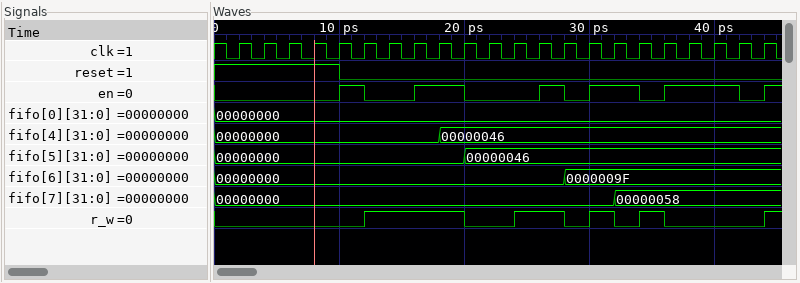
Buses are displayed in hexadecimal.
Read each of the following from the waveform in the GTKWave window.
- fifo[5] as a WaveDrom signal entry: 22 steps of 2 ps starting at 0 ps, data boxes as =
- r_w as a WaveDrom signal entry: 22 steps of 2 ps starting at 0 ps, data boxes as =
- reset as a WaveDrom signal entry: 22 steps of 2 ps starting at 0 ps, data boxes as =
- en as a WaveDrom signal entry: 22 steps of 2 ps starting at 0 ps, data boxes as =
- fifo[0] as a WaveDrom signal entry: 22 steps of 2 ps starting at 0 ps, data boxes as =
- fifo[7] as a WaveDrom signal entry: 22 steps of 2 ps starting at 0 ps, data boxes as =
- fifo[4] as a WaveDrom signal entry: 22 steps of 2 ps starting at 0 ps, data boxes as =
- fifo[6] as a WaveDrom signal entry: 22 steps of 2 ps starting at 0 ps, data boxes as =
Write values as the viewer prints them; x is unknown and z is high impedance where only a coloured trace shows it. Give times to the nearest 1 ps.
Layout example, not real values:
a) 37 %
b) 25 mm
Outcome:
a) {name: 'fifo[5]', wave: '=.........=...........', data: '00000000 00000046'}
b) {name: 'r_w', wave: '0.....1...0.1.01010...'}
c) {name: 'reset', wave: '1....0................'}
d) {name: 'en', wave: '0....10.1.0..101.01..0'}
e) {name: 'fifo[0]', wave: '=.....................', data: '00000000'}
f) {name: 'fifo[7]', wave: '=...............=.....', data: '00000000 00000058'}
g) {name: 'fifo[4]', wave: '=........=............', data: '00000000 00000046'}
h) {name: 'fifo[6]', wave: '=.............=.......', data: '00000000 0000009F'}
